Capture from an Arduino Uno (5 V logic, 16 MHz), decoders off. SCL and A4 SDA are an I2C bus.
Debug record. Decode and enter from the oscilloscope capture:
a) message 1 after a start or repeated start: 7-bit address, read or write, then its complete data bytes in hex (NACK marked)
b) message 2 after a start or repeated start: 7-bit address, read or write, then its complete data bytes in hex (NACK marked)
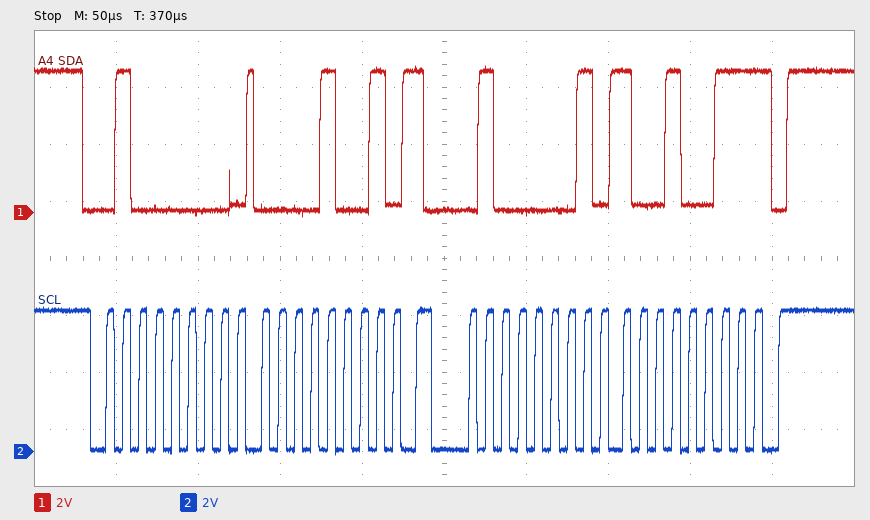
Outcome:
0x20 write: 09
0x20 read: 93 NACK
